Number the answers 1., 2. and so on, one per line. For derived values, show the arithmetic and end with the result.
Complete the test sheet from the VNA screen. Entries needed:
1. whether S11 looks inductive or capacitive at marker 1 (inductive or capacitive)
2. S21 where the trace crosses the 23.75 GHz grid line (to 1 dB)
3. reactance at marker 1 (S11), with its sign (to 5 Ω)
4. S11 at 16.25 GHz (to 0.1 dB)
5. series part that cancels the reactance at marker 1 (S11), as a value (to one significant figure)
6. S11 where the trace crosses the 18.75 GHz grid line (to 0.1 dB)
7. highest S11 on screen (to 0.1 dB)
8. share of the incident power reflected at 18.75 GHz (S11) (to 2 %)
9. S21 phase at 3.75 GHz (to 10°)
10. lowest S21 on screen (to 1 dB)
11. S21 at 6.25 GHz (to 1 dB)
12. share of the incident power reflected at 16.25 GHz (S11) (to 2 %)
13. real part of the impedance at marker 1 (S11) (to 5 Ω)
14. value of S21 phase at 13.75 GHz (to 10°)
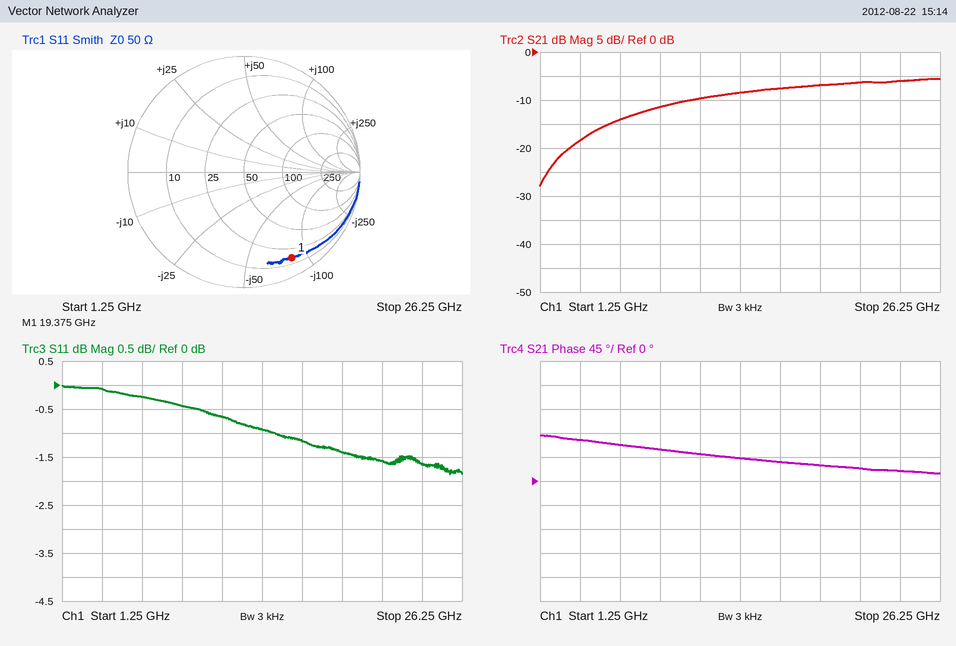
1. capacitive
2. -6 dB
3. -85 Ω
4. -1.2 dB
5. L = 85 Ω/(2π × 19.375 GHz) ≈ 698 pH, so 700 pH to one significant figure
6. -1.4 dB
7. 0.0 dB
8. 10^(-1.4/10) ≈ 72 %
9. 80°
10. -28 dB
11. -14 dB
12. 10^(-1.2/10) ≈ 76 %
13. 15 Ω
14. 40°
